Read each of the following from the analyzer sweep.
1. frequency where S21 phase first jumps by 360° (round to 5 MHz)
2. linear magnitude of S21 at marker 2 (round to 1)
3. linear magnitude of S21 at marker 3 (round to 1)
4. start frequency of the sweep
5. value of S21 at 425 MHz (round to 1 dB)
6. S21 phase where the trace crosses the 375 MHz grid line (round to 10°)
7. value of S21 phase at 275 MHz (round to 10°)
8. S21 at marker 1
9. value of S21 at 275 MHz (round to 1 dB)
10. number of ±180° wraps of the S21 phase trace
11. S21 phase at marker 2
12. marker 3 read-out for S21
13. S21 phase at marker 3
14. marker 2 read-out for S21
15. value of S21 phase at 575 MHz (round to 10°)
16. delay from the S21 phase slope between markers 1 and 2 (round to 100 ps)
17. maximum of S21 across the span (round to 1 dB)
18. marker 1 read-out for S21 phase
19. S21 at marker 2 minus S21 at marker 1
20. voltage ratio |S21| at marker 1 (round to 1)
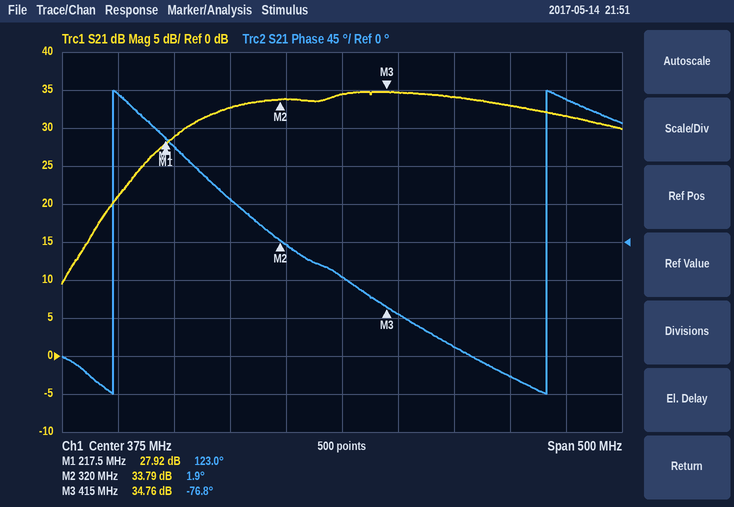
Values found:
170 MHz
49
55
125 MHz
35 dB
-40°
50°
27.92 dB
33 dB
2
1.9°
34.76 dB
-76.8°
33.79 dB
170°
3.3 ns
35 dB
123.0°
5.87 dB
25
